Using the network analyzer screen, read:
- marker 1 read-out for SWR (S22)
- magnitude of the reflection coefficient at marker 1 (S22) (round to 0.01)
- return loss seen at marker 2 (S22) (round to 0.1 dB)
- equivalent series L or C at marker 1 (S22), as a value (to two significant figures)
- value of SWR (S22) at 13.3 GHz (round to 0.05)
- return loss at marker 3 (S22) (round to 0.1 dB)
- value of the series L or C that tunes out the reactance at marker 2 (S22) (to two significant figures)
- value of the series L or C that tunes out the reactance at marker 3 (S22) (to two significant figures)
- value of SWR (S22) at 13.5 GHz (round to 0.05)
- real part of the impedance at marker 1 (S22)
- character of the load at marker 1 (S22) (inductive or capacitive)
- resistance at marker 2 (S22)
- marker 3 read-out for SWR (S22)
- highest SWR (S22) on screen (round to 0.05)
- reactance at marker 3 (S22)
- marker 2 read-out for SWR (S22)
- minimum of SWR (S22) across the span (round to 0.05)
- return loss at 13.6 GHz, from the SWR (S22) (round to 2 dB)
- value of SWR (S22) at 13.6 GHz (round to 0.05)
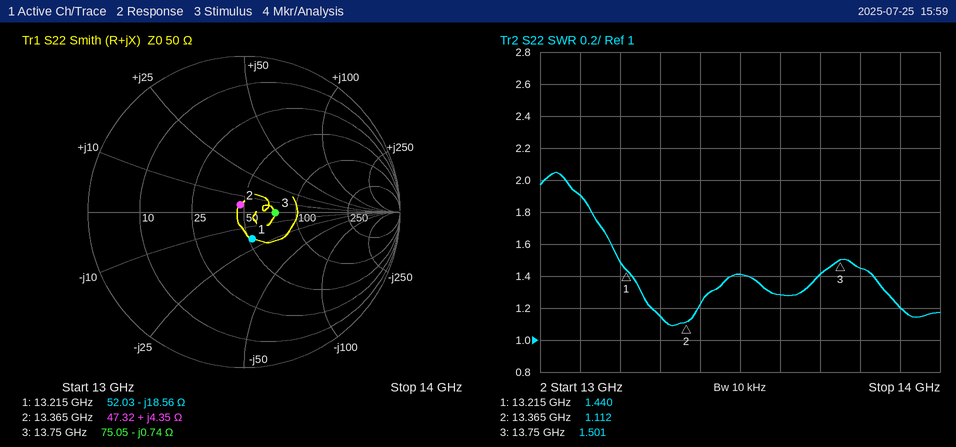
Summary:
1.440
0.18
25.6 dB
650 fF
1.15
14.0 dB
2.7 pF
8.6 pH
1.40
52.03 Ω
capacitive
47.32 Ω
1.501
2.05
-0.74 Ω
1.112
1.10
18 dB
1.30
